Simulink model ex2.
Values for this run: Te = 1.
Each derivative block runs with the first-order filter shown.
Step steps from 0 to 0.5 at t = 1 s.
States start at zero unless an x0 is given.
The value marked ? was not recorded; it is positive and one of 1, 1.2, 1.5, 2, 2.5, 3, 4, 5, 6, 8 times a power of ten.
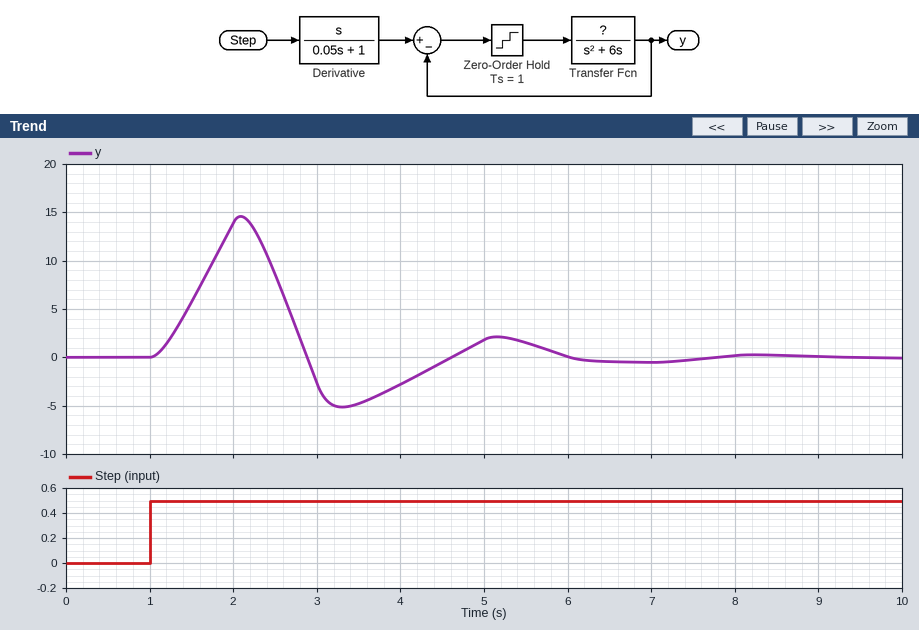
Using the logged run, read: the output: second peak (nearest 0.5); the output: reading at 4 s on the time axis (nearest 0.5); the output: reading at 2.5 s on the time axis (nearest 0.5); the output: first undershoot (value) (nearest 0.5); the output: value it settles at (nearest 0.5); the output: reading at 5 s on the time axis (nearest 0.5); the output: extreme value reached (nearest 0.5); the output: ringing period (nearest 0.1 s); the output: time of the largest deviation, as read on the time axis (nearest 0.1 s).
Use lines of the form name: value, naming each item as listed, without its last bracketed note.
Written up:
the output: second peak: 2.0
the output: reading at 4 s on the time axis: -3.0
the output: reading at 2.5 s on the time axis: 8.5
the output: first undershoot (value): -5.0
the output: value it settles at: 0.0
the output: reading at 5 s on the time axis: 2.0
the output: extreme value reached: 14.5
the output: ringing period: 3.1 s
the output: time of the largest deviation, as read on the time axis: 2.1 s
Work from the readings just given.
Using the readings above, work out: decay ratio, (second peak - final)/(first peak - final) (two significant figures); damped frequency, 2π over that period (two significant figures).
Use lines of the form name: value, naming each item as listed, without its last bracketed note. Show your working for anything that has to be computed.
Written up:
decay ratio, (second peak - final)/(first peak - final): (2 - 0) / (14.5 - 0) = 0.14
damped frequency, 2π over that period: 2π / 3.1 = 2.0 rad/s
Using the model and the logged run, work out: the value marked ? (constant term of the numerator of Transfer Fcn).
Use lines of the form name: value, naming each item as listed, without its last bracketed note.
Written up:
the value marked ?: 10
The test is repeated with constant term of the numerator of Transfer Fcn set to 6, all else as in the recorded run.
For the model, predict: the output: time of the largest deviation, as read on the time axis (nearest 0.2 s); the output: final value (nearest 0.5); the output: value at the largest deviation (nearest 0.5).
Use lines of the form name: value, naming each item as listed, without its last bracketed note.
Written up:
the output: time of the largest deviation, as read on the time axis: 2.2 s
the output: final value: 0.0
the output: value at the largest deviation: 9.0
